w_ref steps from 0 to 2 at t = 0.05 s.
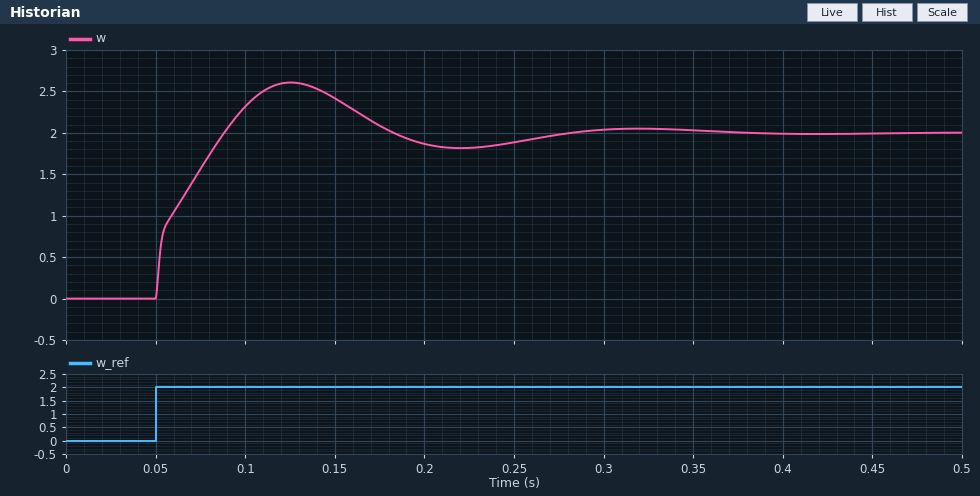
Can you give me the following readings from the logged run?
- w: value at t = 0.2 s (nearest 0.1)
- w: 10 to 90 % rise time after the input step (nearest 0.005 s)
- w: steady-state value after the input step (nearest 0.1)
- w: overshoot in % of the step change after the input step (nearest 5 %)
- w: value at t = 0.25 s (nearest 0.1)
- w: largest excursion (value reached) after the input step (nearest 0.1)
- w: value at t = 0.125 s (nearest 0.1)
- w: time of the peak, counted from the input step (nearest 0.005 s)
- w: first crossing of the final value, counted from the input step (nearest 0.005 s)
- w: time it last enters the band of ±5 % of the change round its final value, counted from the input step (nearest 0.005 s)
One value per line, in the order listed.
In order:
1.9
0.030 s
2.0
30 %
1.9
2.6
2.6
0.075 s
0.040 s
0.205 s
